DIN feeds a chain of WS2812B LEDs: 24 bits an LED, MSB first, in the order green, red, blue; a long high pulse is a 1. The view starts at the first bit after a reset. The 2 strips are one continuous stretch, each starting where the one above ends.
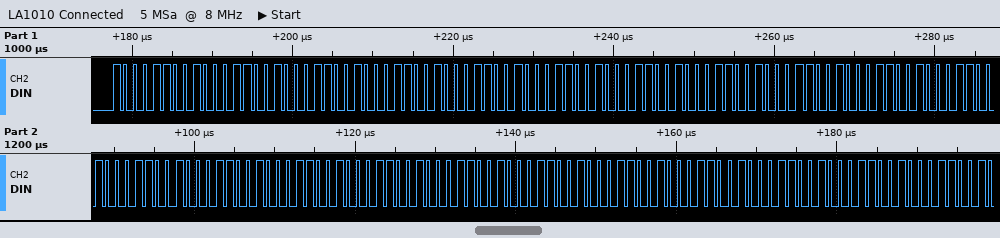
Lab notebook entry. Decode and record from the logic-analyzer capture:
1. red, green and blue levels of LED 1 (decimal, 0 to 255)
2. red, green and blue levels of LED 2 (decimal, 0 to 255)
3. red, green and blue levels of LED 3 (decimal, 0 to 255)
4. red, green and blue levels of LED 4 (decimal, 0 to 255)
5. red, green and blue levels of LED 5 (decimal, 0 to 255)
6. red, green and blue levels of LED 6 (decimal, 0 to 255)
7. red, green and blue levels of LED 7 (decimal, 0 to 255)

140, 140, 140
140, 140, 140
140, 140, 140
140, 140, 140
140, 140, 140
140, 140, 140
140, 140, 140
